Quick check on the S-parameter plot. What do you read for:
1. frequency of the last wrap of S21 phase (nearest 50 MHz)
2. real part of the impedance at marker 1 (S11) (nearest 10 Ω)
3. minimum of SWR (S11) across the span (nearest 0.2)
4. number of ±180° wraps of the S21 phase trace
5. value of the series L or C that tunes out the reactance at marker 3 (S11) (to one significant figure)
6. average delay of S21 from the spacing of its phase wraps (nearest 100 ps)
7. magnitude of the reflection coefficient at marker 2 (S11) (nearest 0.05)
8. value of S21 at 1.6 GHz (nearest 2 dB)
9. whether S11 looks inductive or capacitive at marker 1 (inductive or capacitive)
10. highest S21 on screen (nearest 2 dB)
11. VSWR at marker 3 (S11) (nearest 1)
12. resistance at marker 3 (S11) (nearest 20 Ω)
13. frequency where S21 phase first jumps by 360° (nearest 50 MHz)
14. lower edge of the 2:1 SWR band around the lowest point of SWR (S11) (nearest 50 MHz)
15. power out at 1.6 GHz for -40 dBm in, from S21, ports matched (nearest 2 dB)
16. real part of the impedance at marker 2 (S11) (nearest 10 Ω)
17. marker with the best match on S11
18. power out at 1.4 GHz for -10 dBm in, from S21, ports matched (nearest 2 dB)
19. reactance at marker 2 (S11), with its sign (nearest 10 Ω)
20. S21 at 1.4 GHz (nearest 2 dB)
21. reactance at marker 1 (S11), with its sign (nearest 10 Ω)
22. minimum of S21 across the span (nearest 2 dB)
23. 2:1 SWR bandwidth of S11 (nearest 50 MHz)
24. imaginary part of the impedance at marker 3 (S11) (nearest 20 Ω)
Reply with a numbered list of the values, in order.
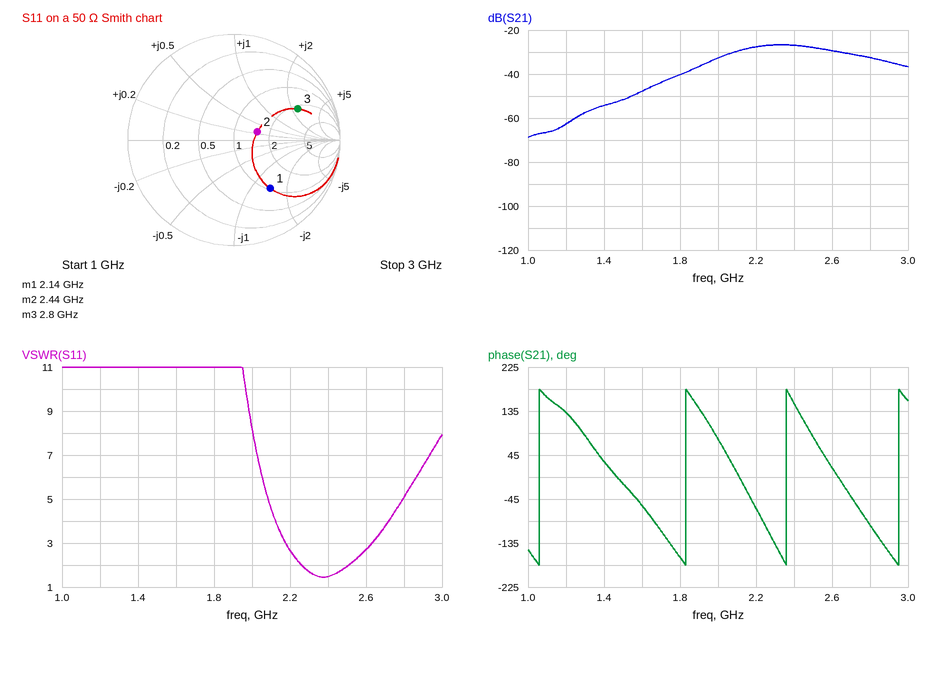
1. 2.95 GHz
2. 50 Ω
3. 1.4
4. 4
5. 500 fF
6. 1.6 ns
7. 0.25
8. -48 dB
9. capacitive
10. -26 dB
11. 5
12. 120 Ω
13. 1.05 GHz
14. 2.25 GHz
15. -88 dBm
16. 80 Ω
17. marker 2
18. -64 dBm
19. +10 Ω
20. -54 dB
21. -70 Ω
22. -68 dB
23. 250 MHz
24. +120 Ω
